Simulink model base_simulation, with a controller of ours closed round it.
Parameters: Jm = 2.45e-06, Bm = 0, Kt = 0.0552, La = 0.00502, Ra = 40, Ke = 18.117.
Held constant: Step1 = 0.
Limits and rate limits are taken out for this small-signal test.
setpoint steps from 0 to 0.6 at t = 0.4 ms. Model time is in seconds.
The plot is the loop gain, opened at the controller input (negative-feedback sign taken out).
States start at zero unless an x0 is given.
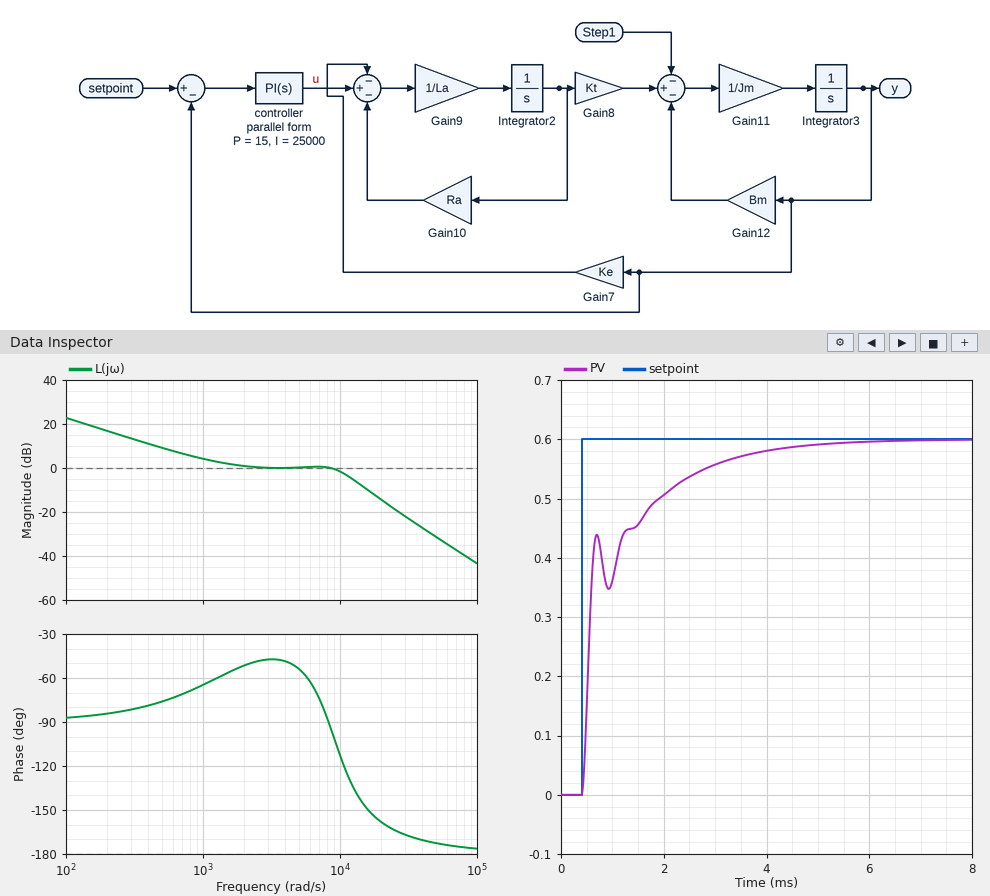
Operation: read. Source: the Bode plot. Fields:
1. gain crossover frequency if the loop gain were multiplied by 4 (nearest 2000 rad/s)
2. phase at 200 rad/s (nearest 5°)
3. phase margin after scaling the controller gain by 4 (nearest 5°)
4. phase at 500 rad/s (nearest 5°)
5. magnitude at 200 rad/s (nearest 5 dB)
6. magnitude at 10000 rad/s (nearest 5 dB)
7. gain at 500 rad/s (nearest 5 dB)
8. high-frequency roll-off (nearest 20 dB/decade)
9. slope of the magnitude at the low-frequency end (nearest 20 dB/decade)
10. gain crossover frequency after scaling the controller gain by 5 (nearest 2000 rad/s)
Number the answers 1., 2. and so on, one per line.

1. 18000 rad/s
2. -85°
3. 25°
4. -75°
5. 15 dB
6. 0 dB
7. 10 dB
8. -40 dB/decade
9. -20 dB/decade
10. 20000 rad/s
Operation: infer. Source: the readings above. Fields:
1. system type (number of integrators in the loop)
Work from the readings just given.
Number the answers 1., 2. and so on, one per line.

1. 1
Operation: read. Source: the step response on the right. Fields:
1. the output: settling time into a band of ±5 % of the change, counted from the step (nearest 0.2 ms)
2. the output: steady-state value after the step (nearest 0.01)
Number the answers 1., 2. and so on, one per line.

1. 3.0 ms
2. 0.60
